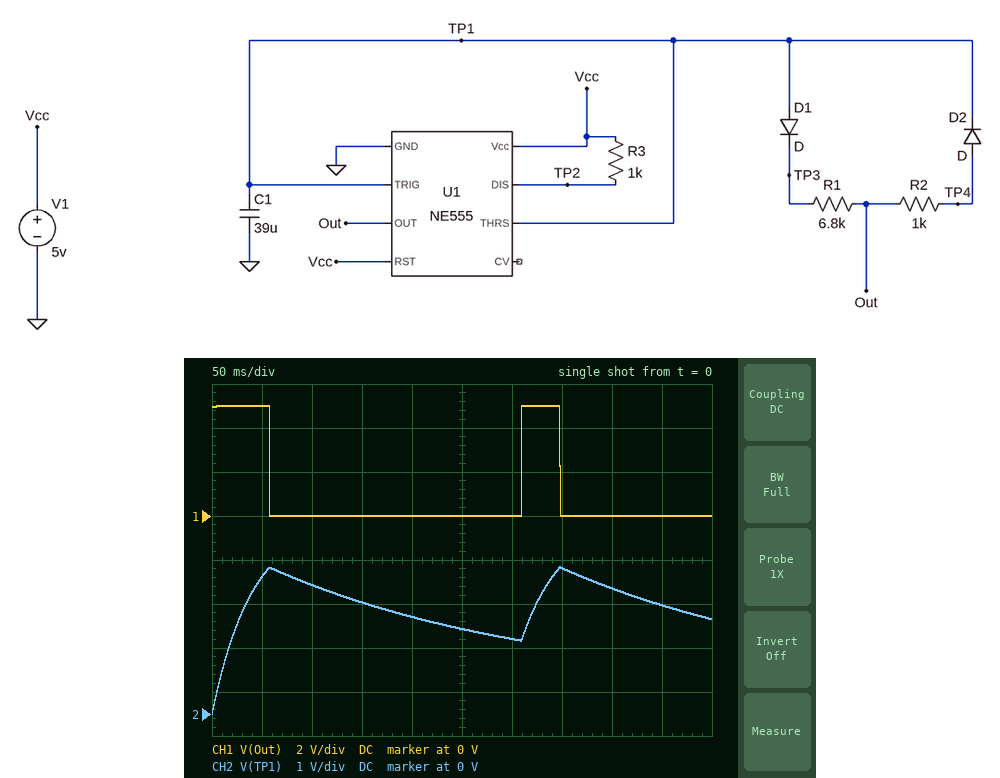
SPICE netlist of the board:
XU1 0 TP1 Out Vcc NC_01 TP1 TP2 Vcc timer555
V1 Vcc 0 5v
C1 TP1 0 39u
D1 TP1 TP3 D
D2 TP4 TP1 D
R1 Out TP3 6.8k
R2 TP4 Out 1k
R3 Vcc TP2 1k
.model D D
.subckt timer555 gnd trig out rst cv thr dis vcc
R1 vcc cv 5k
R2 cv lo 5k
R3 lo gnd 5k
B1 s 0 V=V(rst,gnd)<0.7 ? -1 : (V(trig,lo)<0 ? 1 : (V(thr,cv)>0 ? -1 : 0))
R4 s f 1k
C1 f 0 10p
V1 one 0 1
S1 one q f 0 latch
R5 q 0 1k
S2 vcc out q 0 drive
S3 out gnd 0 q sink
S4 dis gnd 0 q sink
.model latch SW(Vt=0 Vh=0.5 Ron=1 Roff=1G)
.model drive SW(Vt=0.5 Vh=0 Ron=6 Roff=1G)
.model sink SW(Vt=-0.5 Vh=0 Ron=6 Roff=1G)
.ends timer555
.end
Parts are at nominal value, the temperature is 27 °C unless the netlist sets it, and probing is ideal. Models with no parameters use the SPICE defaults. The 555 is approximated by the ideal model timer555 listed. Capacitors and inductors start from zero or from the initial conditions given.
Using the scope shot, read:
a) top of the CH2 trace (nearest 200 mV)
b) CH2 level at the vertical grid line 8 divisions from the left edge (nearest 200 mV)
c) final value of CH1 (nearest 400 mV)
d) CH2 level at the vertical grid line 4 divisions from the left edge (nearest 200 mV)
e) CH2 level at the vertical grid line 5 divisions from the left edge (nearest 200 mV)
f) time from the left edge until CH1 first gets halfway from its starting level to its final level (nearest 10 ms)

3.4 V
2.8 V
0 V
2.2 V
2.0 V
60 ms
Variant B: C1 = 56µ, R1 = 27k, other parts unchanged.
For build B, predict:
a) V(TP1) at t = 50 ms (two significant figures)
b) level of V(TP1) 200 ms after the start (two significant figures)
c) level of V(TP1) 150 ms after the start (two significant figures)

2.5 V
3.1 V
3.2 V
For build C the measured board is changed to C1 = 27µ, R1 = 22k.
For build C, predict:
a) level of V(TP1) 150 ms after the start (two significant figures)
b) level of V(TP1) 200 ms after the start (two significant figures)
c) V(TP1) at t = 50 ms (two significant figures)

2.9 V
2.7 V
3.3 V
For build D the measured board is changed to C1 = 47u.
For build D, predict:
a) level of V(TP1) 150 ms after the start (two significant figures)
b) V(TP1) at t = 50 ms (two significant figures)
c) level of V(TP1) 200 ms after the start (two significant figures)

2.7 V
2.8 V
2.4 V
